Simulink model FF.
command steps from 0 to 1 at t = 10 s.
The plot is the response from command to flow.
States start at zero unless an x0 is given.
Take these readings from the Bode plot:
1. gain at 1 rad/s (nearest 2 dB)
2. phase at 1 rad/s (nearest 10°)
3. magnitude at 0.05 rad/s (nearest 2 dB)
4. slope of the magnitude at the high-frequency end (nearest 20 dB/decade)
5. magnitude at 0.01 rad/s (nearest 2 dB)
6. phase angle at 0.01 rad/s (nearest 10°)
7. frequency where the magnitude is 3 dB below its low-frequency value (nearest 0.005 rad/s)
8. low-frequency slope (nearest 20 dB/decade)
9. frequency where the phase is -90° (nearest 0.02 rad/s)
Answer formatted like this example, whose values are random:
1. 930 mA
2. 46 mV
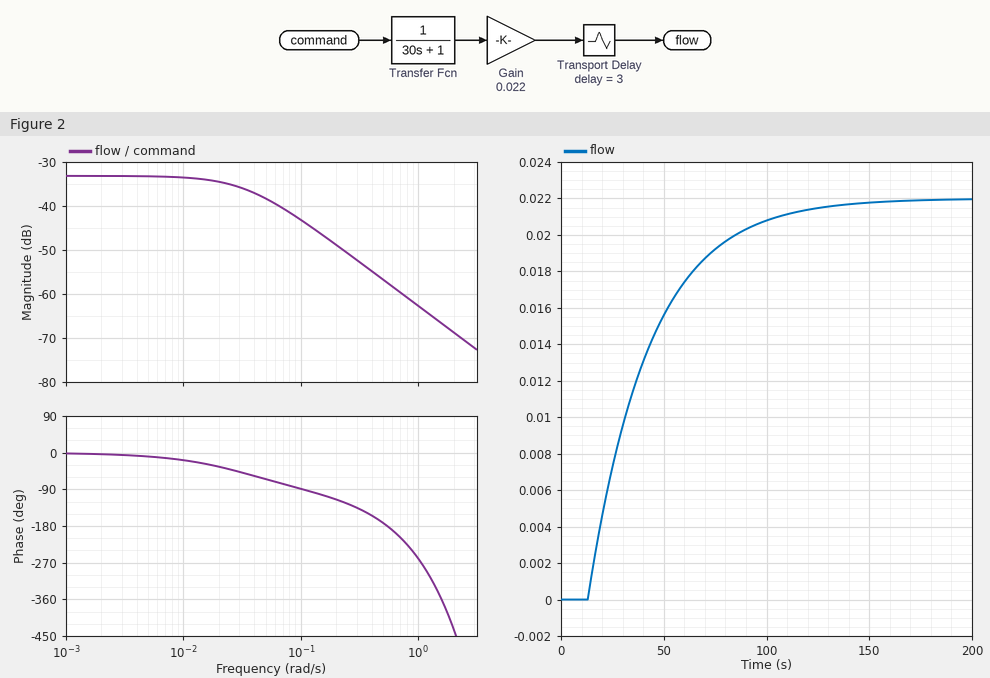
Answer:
1. -62 dB
2. -260°
3. -38 dB
4. -20 dB/decade
5. -34 dB
6. -20°
7. 0.035 rad/s
8. 0 dB/decade
9. 0.10 rad/s
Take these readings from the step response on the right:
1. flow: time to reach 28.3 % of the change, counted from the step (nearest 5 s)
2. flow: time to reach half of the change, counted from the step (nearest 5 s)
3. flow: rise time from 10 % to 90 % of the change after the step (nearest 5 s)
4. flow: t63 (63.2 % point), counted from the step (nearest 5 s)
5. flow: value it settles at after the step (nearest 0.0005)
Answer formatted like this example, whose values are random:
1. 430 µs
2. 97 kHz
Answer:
1. 15 s
2. 25 s
3. 65 s
4. 35 s
5. 0.0220
